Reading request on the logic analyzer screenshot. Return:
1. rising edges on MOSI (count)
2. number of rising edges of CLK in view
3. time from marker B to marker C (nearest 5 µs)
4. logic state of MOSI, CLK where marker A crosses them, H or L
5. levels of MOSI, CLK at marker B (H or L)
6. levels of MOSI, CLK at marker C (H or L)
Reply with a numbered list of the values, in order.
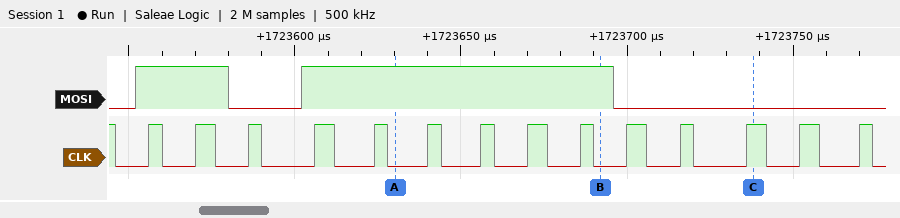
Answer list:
1. 2
2. 14
3. 45 µs
4. MOSI=H, CLK=L
5. MOSI=H, CLK=L
6. MOSI=L, CLK=H
